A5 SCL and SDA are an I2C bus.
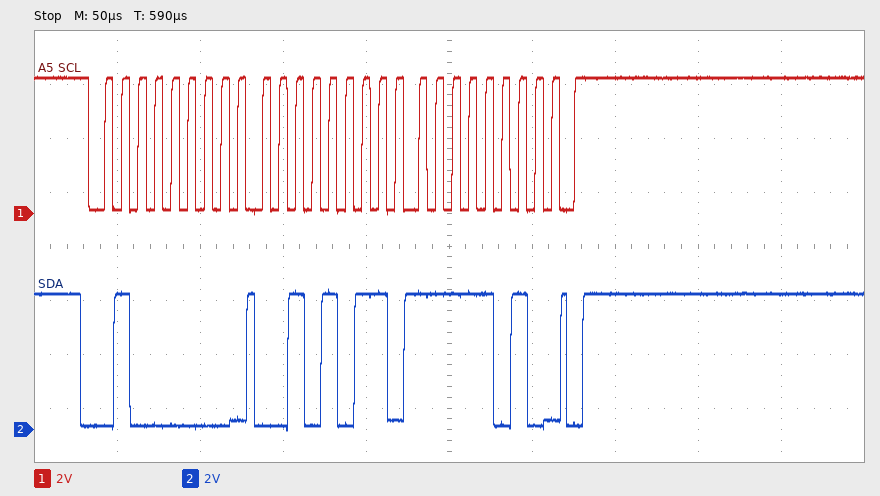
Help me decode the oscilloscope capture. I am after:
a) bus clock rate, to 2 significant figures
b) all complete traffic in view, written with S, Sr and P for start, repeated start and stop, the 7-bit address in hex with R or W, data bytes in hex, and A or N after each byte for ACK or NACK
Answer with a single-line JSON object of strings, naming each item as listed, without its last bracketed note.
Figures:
{"bus clock rate, to 2 significant figures": "100 kHz", "all complete traffic in view, written with S, Sr and P for start, repeated start and stop, the 7-bit address in hex with R or W, data bytes in hex, and A or N after each byte for ACK or NACK": "S 20W A 2B A FA A P"}
